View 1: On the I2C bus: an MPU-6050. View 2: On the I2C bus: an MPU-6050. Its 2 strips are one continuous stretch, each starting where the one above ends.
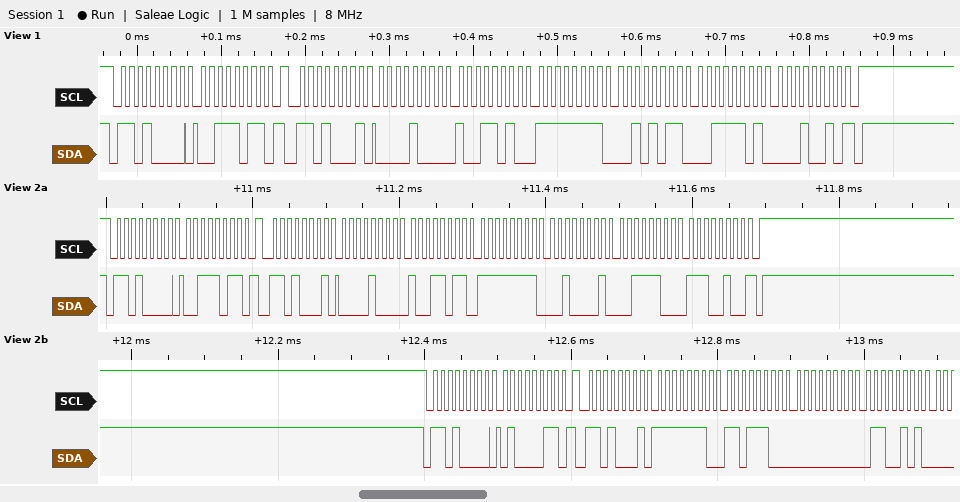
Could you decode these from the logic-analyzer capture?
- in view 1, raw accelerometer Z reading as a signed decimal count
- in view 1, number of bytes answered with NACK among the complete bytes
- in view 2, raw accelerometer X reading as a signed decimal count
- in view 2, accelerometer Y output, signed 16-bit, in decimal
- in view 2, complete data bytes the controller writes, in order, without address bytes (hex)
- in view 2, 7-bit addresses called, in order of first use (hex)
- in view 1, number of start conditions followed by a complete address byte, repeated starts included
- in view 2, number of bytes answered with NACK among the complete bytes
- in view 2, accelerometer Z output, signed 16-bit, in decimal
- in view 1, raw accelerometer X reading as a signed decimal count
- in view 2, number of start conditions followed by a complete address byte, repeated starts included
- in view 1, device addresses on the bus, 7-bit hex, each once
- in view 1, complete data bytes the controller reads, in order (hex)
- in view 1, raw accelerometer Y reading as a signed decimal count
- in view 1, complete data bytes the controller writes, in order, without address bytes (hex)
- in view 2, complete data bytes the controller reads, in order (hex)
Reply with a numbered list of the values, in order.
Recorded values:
1. 15634
2. 1
3. 2203
4. -223
5. 3B 43
6. 0x68
7. 2
8. 1
9. 15588
10. 2202
11. 4
12. 0x68
13. 08 9A FF 2B 3D 12
14. -213
15. 3B
16. 08 9B FF 21 3C E4 FE DC 00 65
